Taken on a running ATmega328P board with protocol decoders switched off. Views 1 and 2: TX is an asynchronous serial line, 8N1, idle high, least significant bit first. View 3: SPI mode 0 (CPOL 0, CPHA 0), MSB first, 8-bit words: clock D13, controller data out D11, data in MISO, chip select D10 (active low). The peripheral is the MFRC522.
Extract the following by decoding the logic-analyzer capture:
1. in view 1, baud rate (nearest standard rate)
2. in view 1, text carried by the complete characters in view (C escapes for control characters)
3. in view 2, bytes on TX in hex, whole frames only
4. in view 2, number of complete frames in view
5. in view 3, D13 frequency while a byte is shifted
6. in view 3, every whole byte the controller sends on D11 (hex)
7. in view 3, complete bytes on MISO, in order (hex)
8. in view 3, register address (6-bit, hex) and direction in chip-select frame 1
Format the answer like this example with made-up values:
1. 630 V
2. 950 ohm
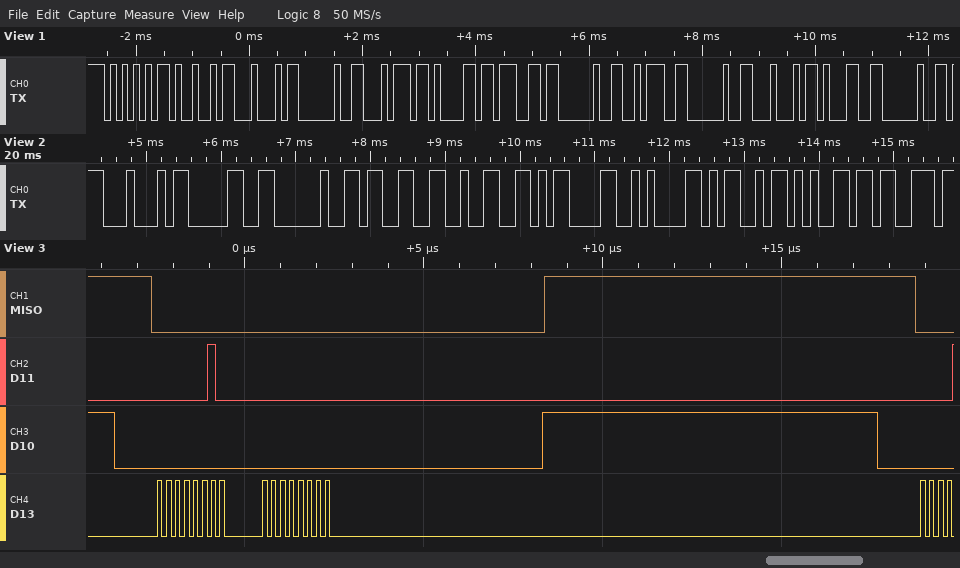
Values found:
1. 9600 baud
2. "UID tag : D1 "
3. 44 30 20 33 32 0D 0A 4D 65 73
4. 10
5. 4 MHz
6. 02 00
7. 00 00
8. 0x01 write
